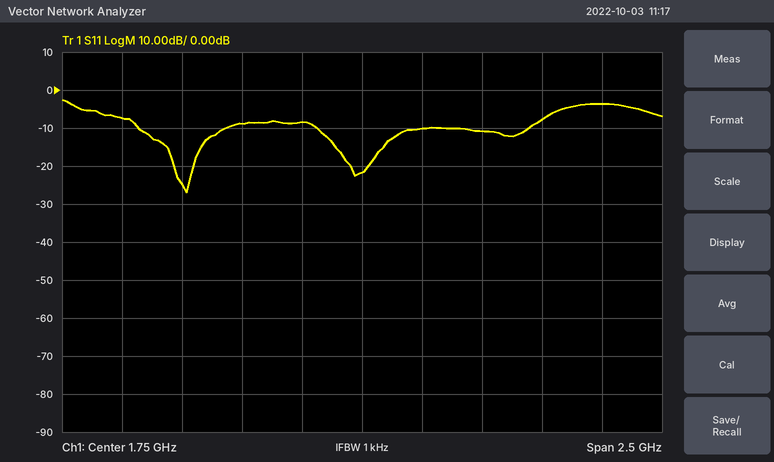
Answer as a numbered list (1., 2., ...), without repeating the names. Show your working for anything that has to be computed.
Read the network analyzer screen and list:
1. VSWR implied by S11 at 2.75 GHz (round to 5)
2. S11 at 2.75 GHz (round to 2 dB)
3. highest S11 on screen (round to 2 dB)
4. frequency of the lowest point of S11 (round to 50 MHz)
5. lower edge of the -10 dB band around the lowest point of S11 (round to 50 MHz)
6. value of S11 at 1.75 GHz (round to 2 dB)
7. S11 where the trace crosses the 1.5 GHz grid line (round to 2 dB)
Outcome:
1. |Γ| = 10^(-4/20) = 0.6310; VSWR = (1 + 0.6310)/(1 − 0.6310) ≈ 4.42, so 5 to the nearest 5
2. -4 dB
3. -2 dB
4. 1.00 GHz
5. 800 MHz
6. -22 dB
7. -8 dB
